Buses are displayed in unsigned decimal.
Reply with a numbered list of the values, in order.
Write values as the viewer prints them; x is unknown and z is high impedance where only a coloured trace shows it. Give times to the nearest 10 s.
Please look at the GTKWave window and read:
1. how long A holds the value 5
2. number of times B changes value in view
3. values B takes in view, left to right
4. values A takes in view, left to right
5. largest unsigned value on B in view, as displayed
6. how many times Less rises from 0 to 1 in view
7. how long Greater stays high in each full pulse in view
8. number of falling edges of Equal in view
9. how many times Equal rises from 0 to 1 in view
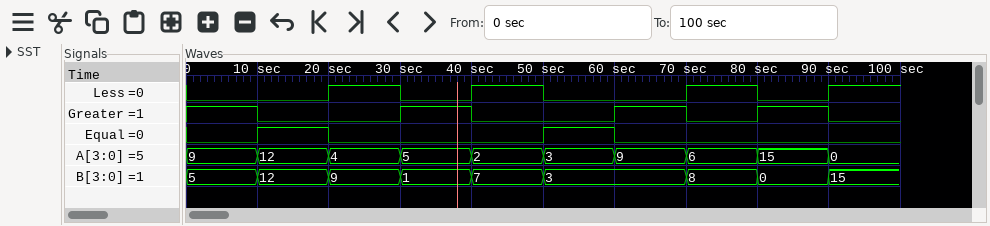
1. 10 s
2. 8
3. 5, 12, 9, 1, 7, 3, 8, 0, 15
4. 9, 12, 4, 5, 2, 3, 9, 6, 15, 0
5. 15
6. 4
7. 10 s, 10 s, 10 s
8. 2
9. 2
